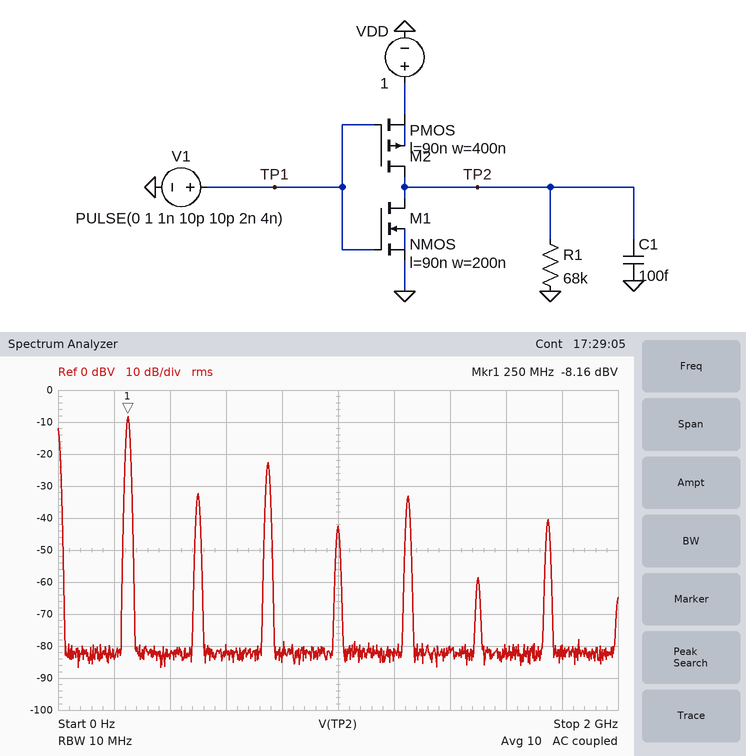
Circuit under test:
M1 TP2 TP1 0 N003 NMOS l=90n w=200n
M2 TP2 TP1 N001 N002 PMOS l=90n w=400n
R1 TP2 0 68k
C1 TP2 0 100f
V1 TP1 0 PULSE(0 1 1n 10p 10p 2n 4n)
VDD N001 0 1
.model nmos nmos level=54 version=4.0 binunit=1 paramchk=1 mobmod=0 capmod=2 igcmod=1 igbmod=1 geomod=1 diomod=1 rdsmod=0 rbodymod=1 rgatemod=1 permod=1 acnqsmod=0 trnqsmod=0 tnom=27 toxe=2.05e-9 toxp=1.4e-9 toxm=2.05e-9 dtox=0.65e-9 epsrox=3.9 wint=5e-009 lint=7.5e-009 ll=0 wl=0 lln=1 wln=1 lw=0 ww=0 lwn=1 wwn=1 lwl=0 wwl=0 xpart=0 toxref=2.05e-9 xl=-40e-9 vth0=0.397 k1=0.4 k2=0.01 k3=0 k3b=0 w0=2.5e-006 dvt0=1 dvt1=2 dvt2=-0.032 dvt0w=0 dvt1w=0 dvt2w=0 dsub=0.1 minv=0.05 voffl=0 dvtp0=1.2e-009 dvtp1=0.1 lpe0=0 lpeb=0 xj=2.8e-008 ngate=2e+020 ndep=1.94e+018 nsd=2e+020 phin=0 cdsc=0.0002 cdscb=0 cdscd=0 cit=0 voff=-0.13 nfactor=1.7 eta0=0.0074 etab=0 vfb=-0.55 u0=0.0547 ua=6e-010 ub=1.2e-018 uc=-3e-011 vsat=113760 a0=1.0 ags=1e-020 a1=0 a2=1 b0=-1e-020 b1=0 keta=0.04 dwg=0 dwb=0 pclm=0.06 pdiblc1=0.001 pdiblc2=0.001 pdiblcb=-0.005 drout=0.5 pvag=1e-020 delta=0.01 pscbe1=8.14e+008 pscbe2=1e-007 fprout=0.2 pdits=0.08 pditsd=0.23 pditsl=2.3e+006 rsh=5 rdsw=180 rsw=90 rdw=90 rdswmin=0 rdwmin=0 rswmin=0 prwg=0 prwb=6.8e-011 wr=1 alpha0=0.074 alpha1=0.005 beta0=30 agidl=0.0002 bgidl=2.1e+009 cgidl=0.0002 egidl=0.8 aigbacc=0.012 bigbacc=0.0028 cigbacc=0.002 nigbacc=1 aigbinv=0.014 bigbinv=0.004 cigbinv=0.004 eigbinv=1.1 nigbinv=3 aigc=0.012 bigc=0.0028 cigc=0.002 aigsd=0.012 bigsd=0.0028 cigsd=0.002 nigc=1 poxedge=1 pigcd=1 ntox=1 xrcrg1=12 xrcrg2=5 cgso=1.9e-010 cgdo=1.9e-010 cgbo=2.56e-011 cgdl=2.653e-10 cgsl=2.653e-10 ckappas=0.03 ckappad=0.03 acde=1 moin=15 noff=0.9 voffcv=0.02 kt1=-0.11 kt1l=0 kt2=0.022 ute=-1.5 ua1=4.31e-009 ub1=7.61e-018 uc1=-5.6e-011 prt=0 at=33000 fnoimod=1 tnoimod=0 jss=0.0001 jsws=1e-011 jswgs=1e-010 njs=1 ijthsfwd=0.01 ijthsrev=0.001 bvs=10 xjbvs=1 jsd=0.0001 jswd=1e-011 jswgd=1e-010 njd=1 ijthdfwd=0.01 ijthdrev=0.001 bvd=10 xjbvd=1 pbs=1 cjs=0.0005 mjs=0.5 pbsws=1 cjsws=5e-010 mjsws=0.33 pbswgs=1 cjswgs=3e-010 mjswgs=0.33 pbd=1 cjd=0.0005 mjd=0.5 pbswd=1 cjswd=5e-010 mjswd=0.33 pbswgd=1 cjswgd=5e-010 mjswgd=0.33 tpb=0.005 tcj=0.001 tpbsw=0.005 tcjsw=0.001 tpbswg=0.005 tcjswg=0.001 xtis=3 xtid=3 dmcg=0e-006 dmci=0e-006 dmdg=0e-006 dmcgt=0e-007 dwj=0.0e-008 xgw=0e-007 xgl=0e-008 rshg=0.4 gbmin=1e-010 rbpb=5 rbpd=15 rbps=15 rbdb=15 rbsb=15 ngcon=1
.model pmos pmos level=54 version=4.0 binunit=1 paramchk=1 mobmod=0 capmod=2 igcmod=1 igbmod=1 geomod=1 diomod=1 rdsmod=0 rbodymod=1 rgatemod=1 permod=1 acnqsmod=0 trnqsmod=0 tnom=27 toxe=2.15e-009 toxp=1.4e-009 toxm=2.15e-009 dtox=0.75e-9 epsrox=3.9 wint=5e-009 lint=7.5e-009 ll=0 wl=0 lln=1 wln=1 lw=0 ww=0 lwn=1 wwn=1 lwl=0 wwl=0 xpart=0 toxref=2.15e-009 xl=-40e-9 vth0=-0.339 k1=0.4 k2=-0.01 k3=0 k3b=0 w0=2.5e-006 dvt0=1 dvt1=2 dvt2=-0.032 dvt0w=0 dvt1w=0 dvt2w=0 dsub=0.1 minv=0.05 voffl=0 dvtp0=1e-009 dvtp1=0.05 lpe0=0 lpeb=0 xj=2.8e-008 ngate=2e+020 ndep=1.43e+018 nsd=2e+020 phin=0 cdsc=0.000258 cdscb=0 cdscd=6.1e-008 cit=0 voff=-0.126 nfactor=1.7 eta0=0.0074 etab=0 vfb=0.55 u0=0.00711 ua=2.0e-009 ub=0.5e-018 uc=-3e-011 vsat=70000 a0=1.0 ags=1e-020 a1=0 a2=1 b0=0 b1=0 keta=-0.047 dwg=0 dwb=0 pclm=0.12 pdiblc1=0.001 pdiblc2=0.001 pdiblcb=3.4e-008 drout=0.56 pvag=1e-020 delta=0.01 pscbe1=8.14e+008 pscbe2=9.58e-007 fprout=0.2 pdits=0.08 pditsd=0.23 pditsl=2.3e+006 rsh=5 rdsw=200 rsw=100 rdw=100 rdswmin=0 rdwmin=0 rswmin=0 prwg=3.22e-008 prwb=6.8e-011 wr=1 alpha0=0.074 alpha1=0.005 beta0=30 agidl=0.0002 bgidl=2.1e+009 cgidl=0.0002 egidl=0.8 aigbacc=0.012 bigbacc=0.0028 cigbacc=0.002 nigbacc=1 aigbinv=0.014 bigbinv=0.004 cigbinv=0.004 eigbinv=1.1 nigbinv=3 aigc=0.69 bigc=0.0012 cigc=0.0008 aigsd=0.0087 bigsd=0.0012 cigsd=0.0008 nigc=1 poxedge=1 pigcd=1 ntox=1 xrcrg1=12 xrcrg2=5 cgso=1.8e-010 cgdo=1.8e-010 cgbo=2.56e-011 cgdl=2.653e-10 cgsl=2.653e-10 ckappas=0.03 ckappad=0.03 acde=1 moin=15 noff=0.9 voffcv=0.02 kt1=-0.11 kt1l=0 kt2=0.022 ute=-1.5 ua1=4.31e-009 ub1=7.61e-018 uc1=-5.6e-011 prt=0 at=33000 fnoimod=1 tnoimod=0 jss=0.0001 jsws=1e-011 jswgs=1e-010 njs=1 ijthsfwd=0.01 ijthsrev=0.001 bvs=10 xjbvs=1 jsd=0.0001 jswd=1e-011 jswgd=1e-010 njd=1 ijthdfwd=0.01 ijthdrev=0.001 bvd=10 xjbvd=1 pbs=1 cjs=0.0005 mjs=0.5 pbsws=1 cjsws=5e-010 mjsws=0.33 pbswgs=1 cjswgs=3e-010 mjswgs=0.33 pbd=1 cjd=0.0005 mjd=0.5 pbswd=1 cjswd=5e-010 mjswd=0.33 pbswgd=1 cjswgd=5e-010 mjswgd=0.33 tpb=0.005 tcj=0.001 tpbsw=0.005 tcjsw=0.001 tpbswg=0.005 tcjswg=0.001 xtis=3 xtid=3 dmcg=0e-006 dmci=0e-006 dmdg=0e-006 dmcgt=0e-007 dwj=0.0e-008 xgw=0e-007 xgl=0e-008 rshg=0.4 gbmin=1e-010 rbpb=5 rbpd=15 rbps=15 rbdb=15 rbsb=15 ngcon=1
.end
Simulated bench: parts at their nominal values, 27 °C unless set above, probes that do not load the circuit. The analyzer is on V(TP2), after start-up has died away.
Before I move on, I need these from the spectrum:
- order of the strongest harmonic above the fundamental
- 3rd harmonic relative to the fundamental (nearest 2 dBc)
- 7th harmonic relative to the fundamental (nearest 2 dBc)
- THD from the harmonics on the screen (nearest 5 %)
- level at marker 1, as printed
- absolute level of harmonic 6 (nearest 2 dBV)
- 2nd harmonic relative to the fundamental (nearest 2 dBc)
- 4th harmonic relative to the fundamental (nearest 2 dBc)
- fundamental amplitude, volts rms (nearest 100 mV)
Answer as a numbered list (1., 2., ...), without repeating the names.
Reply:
1. 3
2. -14 dBc
3. -32 dBc
4. 20 %
5. -8.16 dBV
6. -58 dBV
7. -24 dBc
8. -34 dBc
9. 400 mV
